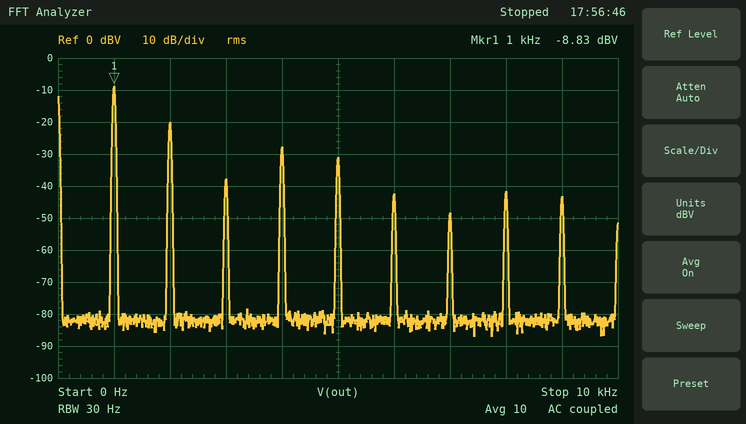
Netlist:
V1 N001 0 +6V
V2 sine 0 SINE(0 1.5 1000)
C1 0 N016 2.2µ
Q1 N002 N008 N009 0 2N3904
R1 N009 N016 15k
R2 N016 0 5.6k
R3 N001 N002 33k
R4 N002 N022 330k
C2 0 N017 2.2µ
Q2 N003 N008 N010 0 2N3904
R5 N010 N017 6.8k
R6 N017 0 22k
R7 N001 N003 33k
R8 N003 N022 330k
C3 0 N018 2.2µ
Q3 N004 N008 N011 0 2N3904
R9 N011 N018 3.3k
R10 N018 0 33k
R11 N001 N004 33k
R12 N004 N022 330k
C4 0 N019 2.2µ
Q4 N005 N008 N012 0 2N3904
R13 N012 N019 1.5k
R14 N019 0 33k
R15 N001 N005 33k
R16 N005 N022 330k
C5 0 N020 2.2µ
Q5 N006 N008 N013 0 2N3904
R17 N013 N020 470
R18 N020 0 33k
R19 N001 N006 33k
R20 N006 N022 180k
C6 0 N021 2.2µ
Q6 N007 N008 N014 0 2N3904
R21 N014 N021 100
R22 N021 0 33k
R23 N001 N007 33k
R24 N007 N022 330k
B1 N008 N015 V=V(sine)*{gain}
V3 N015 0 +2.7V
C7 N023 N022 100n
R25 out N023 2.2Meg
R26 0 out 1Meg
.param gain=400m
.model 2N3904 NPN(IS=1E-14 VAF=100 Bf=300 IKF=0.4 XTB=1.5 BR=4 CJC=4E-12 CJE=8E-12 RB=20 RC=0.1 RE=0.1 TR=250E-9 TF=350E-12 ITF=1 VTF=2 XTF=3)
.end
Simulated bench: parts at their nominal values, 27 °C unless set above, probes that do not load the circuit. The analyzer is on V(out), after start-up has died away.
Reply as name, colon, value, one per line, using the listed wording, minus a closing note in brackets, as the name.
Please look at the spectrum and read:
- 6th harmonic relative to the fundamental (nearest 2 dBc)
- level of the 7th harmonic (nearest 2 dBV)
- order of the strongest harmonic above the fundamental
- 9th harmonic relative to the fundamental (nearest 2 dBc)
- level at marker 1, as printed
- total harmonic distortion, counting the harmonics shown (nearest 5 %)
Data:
6th harmonic relative to the fundamental: -34 dBc
level of the 7th harmonic: -48 dBV
order of the strongest harmonic above the fundamental: 2
9th harmonic relative to the fundamental: -34 dBc
level at marker 1, as printed: -8.83 dBV
total harmonic distortion, counting the harmonics shown: 30 %
